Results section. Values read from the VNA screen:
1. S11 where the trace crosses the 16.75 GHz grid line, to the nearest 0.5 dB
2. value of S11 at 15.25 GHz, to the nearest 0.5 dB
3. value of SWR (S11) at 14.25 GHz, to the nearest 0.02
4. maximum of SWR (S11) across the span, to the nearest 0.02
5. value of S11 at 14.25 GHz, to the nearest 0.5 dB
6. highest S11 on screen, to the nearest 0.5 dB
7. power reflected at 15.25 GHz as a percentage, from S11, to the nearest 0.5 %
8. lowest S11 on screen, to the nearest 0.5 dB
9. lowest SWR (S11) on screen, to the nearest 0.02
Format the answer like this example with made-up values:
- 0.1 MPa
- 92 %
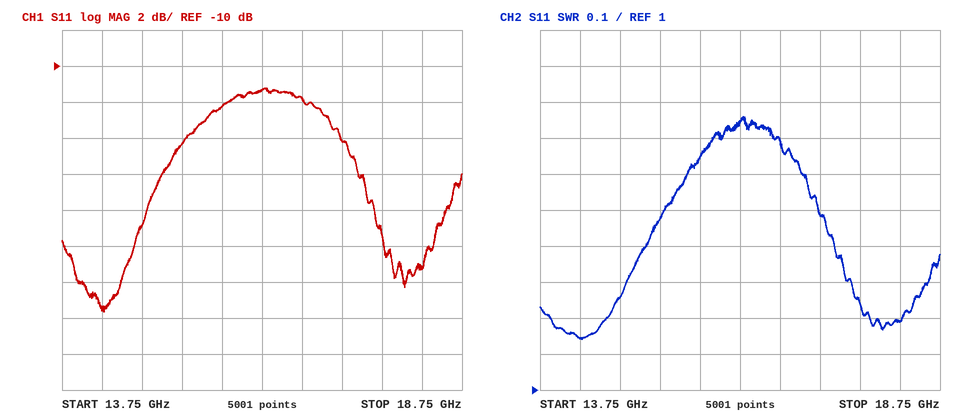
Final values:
- -12.0 dB
- -14.5 dB
- 1.14
- 1.76
- -23.5 dB
- -11.0 dB
- 3.5 %
- -23.5 dB
- 1.14
